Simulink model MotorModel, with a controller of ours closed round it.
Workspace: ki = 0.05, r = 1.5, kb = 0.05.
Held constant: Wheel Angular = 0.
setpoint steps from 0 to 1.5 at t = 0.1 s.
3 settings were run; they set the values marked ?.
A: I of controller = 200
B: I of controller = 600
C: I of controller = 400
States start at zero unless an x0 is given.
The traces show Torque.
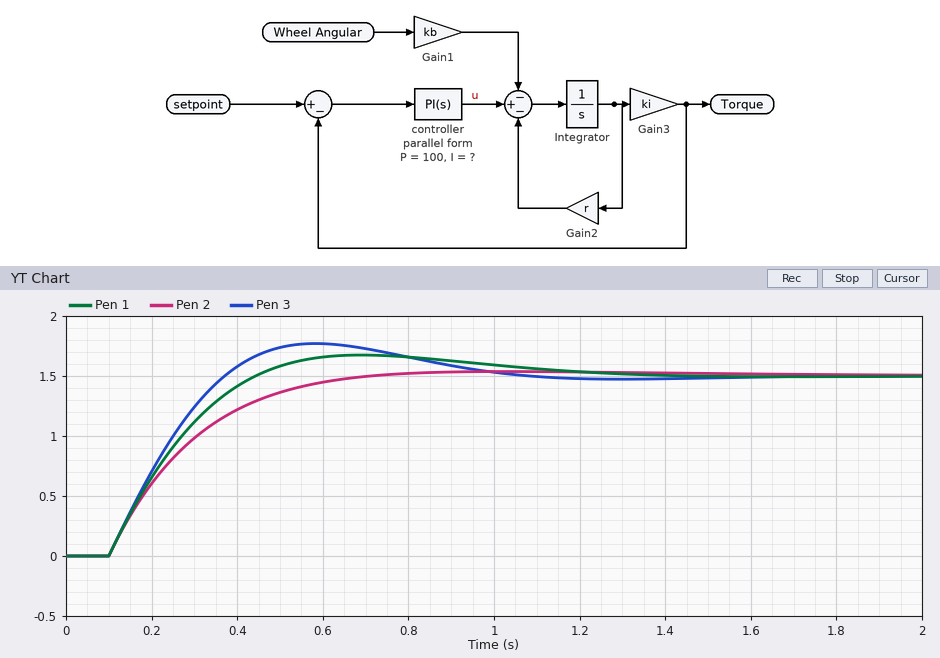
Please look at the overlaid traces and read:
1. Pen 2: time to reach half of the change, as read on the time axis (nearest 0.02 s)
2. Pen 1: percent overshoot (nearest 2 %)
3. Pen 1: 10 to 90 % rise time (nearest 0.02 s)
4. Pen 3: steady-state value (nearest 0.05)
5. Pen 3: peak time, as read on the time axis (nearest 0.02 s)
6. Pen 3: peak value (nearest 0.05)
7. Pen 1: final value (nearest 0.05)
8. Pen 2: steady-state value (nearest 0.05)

0.24 s
12 %
0.26 s
1.50
0.58 s
1.75
1.50
1.50
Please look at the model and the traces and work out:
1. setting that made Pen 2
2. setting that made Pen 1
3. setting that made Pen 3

A
C
B
